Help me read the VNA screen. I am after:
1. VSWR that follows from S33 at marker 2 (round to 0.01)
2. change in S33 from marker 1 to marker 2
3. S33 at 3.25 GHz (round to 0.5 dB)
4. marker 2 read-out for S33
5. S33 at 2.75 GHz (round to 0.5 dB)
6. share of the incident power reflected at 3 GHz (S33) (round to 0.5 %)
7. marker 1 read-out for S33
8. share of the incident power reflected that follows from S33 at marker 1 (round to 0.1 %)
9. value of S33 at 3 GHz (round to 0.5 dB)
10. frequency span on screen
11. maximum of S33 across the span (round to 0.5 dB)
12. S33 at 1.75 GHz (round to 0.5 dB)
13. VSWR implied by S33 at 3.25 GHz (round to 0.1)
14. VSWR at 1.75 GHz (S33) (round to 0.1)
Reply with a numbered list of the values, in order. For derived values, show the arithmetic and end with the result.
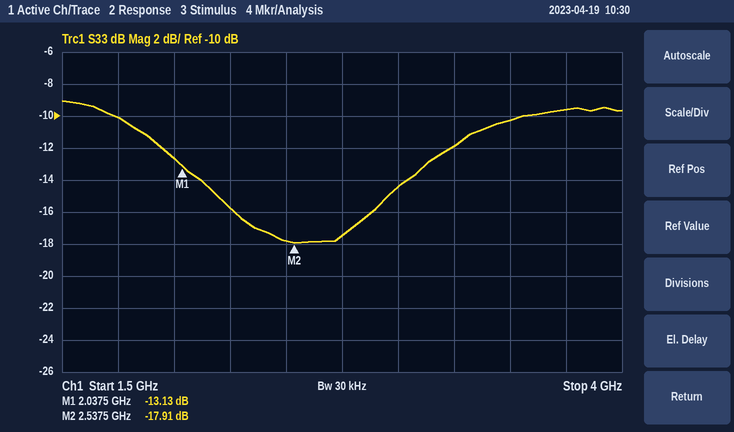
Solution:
1. (1 + 0.1272)/(1 − 0.1272) ≈ 1.29
2. -17.91 − (-13.13) = -4.78 dB
3. -12.0 dB
4. -17.91 dB
5. -17.5 dB
6. 10^(-14.5/10) ≈ 3.5 %
7. -13.13 dB
8. 10^(-13.13/10) ≈ 4.9 %
9. -14.5 dB
10. 2.5 GHz
11. -9.0 dB
12. -10.0 dB
13. |Γ| = 10^(-12/20) = 0.2512; VSWR = (1 + 0.2512)/(1 − 0.2512) ≈ 1.7
14. |Γ| = 10^(-10/20) = 0.3162; VSWR = (1 + 0.3162)/(1 − 0.3162) ≈ 1.9
